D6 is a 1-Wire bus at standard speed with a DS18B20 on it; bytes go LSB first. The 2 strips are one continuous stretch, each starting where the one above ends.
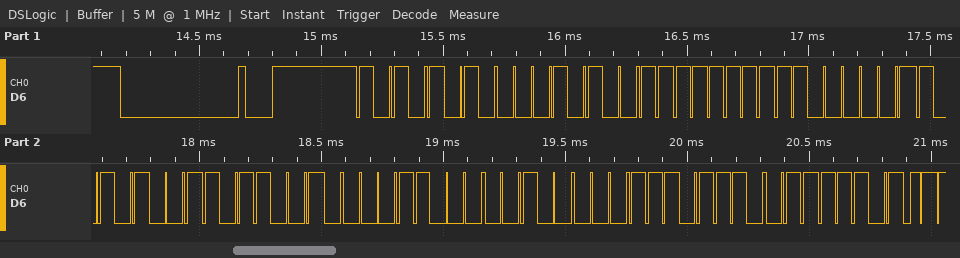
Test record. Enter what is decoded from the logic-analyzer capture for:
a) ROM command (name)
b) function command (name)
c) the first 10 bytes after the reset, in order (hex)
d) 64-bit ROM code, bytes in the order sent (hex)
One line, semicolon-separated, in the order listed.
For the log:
Match ROM; Read Scratchpad; 55 28 FF 83 95 4D 18 04 77 BE; 28 FF 83 95 4D 18 04 77
